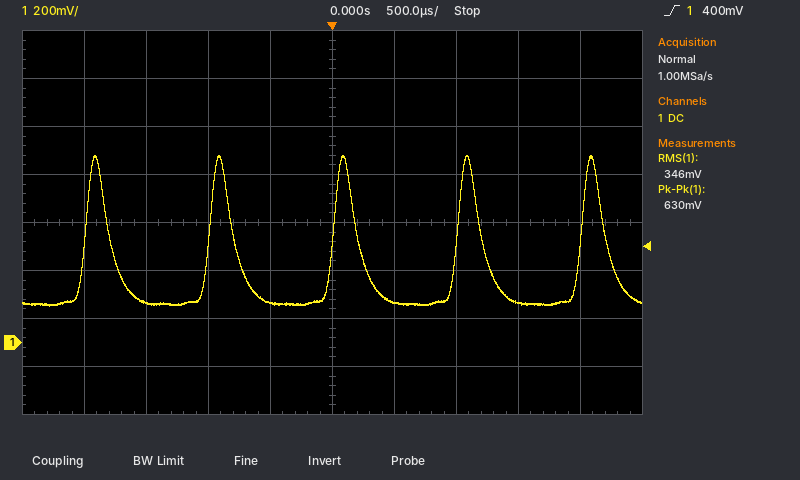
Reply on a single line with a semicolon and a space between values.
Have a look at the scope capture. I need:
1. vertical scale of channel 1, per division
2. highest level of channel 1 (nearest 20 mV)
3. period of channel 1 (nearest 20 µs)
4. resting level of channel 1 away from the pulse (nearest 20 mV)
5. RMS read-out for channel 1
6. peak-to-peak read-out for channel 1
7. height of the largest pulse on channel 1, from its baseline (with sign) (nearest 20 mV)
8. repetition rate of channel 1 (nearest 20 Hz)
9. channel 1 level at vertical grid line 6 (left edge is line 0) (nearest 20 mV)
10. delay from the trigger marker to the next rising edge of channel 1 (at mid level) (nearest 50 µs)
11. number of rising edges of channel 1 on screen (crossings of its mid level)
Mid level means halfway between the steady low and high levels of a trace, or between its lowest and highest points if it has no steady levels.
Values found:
200 mV; 780 mV; 1.00 ms; 160 mV; 346 mV; 630 mV; +620 mV; 1.00 kHz; 160 mV; 1.00 ms; 5
